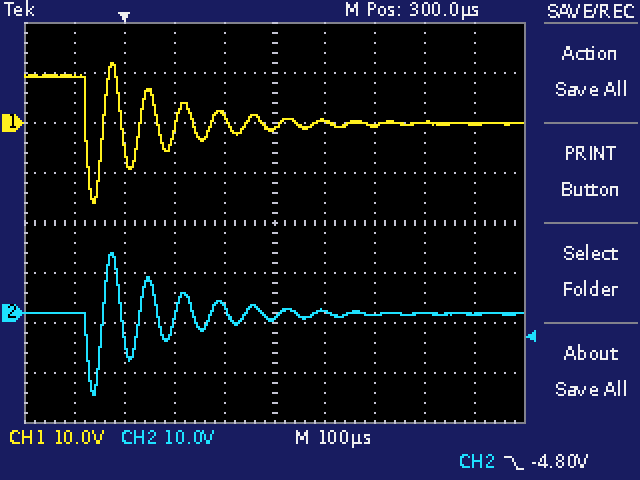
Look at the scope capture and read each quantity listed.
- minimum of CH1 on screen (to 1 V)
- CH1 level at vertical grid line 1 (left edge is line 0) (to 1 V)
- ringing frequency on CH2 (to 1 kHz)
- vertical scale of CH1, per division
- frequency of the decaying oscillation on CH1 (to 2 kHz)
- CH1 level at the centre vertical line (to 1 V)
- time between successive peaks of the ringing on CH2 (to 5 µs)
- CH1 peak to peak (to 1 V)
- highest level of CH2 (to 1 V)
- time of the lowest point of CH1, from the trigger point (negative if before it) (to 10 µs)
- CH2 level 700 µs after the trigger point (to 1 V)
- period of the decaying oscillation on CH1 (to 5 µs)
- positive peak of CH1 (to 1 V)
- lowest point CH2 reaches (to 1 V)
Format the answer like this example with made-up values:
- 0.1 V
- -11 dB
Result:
- -16 V
- 9 V
- 14 kHz
- 10 V
- 14 kHz
- -1 V
- 70 µs
- 28 V
- 12 V
- -60 µs
- 0 V
- 70 µs
- 12 V
- -16 V
